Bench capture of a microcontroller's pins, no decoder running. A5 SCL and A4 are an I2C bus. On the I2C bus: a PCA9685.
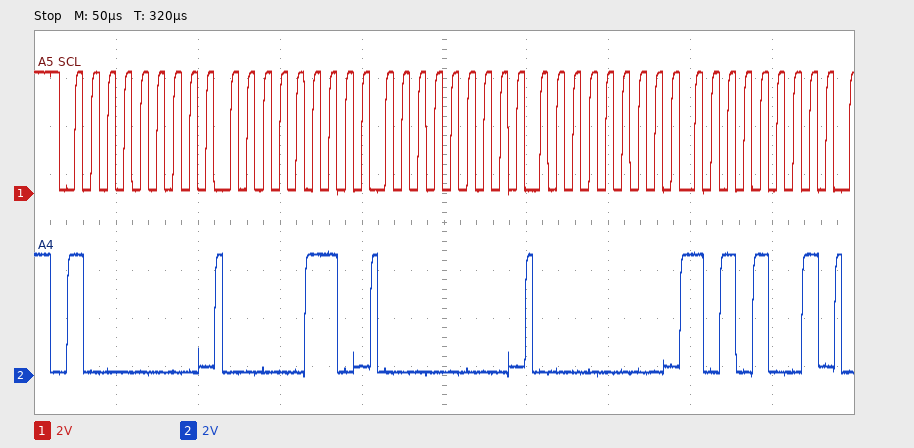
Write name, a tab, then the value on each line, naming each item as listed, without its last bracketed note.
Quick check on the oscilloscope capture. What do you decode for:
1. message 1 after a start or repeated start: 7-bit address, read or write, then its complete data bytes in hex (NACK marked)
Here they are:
message 1 after a start or repeated start: 7-bit address, read or write, then its complete data bytes in hex	0x40 write: 06 00 00 A9
